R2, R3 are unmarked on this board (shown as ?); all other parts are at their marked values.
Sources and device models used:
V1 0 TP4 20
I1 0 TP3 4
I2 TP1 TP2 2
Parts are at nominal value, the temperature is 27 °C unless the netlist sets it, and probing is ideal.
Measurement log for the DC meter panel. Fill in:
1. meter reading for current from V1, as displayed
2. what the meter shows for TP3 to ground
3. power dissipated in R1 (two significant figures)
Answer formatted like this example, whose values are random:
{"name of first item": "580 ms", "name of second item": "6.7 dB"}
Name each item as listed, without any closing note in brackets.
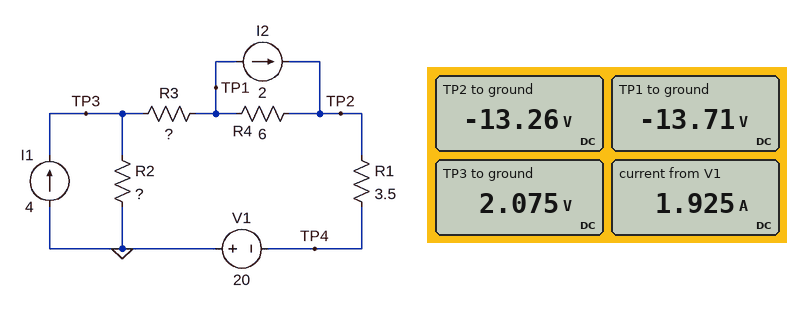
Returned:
{"meter reading for current from V1, as displayed": "1.925 A", "what the meter shows for TP3 to ground": "2.075 V", "power dissipated in R1": "13 W"}
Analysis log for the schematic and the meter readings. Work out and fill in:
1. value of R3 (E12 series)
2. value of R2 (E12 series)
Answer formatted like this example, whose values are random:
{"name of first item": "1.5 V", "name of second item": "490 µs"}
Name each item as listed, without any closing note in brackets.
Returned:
{"value of R3": "8.2 Ω", "value of R2": "1 Ω"}
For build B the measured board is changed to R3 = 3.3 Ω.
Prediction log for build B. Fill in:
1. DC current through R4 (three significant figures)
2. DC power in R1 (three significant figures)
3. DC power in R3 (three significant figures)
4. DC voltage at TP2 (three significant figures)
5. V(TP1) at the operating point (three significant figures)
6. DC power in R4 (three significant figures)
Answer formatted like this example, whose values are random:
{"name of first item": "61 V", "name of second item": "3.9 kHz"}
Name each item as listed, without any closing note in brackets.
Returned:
{"DC current through R4": "609 mA", "DC power in R1": "23.8 W", "DC power in R3": "22.5 W", "DC voltage at TP2": "-10.9 V", "V(TP1) at the operating point": "-7.22 V", "DC power in R4": "2.22 W"}
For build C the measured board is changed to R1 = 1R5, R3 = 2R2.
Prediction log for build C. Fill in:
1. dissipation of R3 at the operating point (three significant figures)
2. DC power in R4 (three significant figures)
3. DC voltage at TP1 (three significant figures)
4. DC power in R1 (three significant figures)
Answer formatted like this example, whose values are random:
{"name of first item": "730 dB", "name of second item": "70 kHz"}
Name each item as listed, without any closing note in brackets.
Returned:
{"dissipation of R3 at the operating point": "24.9 W", "DC power in R4": "11.2 W", "DC voltage at TP1": "-6.77 V", "DC power in R1": "17.0 W"}
